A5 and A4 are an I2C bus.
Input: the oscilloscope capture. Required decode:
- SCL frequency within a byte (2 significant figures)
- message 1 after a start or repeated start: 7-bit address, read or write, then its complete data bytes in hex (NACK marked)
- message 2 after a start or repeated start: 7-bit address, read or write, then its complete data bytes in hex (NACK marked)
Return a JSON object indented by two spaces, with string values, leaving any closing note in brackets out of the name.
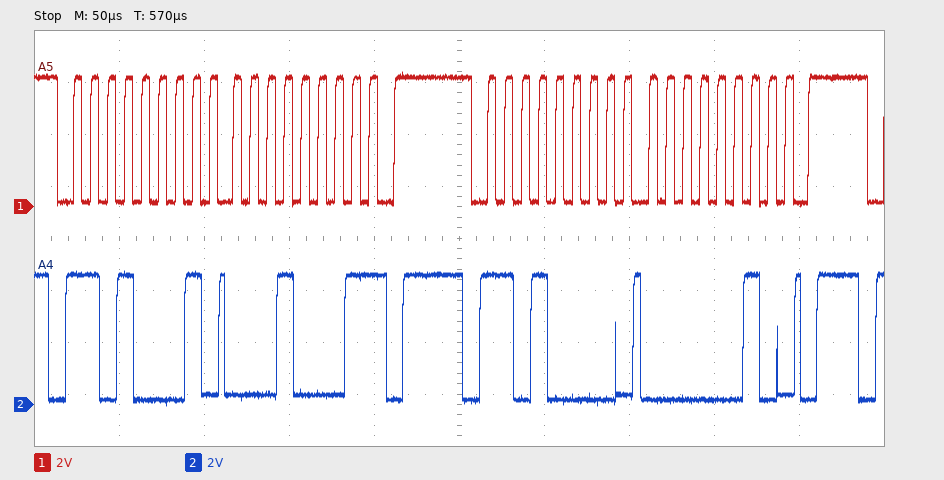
{
  "SCL frequency within a byte": "100 kHz",
  "message 1 after a start or repeated start: 7-bit address, read or write, then its complete data bytes in hex": "0x68 read: 11 NACK",
  "message 2 after a start or repeated start: 7-bit address, read or write, then its complete data bytes in hex": "0x68 write: 02"
}
